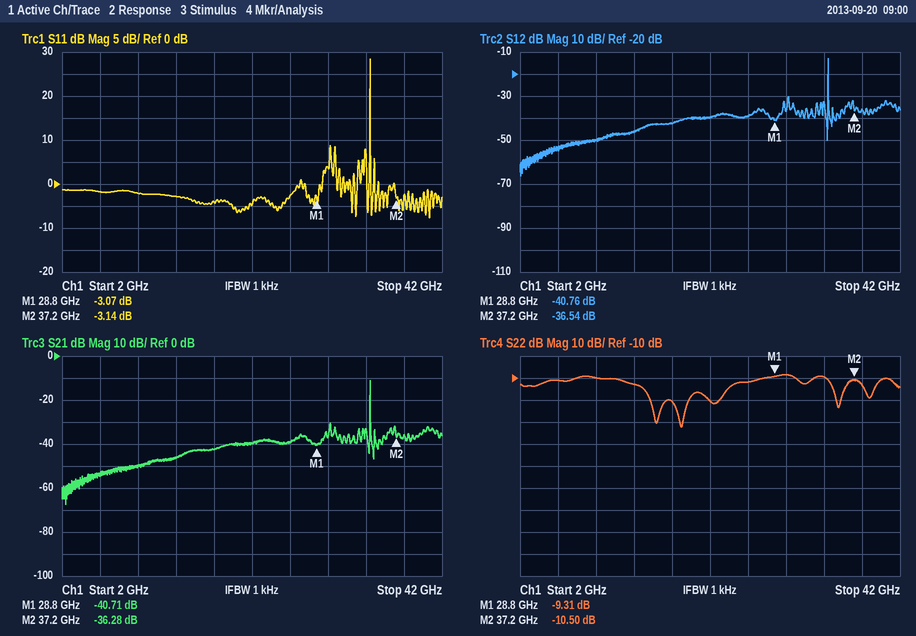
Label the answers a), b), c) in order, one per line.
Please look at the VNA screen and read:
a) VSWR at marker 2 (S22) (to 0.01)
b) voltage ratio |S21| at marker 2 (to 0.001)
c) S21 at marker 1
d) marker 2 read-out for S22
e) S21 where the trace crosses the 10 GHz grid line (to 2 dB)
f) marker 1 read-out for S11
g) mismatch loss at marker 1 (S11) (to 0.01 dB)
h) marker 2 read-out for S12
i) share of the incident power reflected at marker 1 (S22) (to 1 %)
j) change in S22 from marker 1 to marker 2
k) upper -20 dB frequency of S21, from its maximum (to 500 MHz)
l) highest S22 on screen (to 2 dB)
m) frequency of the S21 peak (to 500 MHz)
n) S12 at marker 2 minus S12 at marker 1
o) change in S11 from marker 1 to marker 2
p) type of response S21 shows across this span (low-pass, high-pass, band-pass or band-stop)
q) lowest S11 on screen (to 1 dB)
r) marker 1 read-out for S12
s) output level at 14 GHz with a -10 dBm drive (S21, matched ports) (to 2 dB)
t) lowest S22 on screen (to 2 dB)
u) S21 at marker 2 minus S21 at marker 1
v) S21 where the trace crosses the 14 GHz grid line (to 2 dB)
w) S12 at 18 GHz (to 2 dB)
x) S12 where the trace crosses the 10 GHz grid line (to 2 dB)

a) 1.85
b) 0.015
c) -40.71 dB
d) -10.50 dB
e) -50 dB
f) -3.07 dB
g) 2.95 dB
h) -36.54 dB
i) 12 %
j) -1.19 dB
k) 34.5 GHz
l) -8 dB
m) 34.5 GHz
n) 4.22 dB
o) -0.07 dB
p) band-pass
q) -8 dB
r) -40.76 dB
s) -56 dBm
t) -32 dB
u) 4.43 dB
v) -46 dB
w) -42 dB
x) -50 dB
